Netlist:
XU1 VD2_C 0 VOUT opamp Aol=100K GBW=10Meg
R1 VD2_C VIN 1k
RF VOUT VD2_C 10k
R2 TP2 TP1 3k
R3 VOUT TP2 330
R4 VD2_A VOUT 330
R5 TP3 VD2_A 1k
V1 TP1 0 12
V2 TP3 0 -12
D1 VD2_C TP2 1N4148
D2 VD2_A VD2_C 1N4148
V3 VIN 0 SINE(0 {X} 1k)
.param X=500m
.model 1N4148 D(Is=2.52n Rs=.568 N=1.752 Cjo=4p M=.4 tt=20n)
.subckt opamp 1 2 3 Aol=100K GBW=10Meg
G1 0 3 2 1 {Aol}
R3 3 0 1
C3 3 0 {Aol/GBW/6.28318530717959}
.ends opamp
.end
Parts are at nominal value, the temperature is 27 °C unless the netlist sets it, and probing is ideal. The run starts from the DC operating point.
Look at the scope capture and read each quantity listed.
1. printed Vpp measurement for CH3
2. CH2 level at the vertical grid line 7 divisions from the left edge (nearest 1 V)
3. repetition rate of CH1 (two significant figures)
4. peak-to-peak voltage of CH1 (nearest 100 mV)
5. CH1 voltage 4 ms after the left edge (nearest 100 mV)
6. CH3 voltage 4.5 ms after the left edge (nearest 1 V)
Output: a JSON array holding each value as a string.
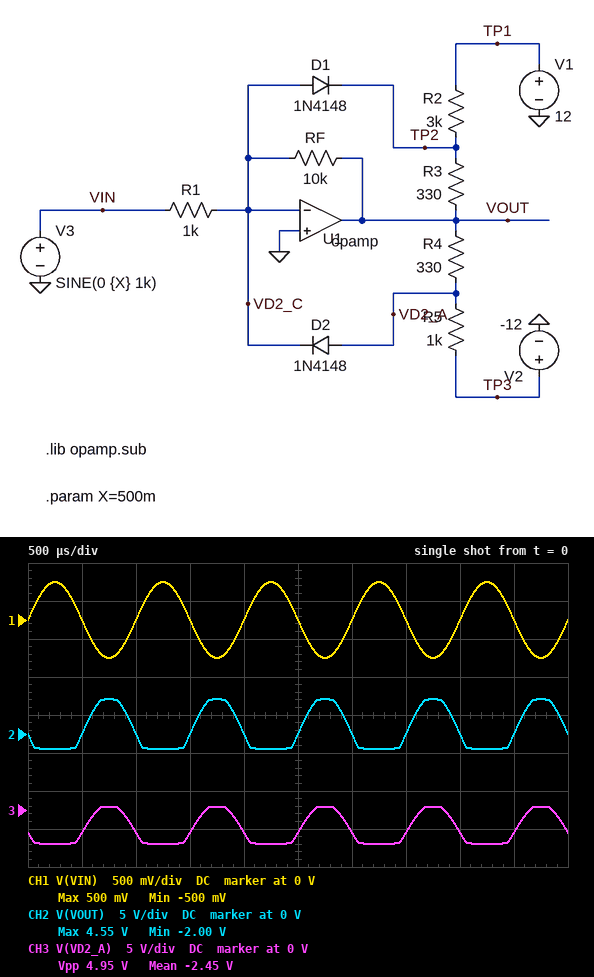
["4.95 V", "0 V", "1.0 kHz", "1.0 V", "0 V", "-3 V"]
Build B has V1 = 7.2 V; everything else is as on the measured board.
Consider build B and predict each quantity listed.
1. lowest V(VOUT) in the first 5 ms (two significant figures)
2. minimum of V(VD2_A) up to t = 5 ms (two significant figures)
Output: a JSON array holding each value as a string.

["-1.5 V", "-4.1 V"]
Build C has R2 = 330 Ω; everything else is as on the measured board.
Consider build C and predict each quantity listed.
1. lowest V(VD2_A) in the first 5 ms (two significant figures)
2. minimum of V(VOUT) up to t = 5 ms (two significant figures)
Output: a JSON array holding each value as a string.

["-6.7 V", "-5.0 V"]
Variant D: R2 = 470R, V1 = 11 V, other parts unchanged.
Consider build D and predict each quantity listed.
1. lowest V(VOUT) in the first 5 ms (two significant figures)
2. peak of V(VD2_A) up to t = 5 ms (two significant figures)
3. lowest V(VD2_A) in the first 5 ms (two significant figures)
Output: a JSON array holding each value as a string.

["-5.0 V", "440 mV", "-6.7 V"]
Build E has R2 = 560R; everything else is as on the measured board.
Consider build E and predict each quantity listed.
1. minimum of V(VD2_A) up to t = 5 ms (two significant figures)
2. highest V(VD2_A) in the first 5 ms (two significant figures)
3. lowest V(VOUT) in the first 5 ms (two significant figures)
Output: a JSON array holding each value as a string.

["-6.7 V", "440 mV", "-5.0 V"]
